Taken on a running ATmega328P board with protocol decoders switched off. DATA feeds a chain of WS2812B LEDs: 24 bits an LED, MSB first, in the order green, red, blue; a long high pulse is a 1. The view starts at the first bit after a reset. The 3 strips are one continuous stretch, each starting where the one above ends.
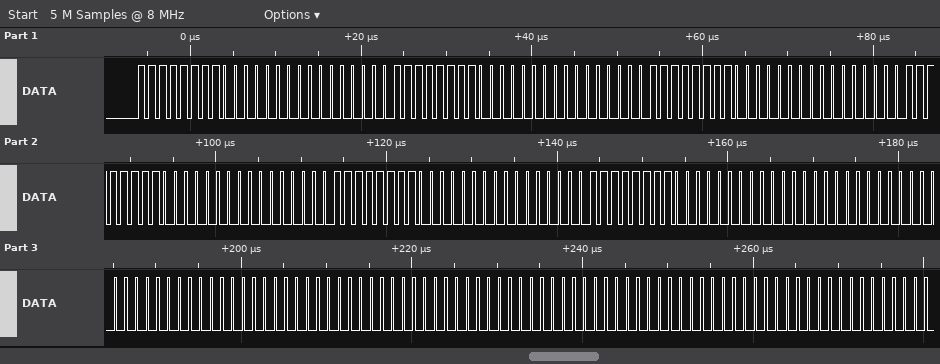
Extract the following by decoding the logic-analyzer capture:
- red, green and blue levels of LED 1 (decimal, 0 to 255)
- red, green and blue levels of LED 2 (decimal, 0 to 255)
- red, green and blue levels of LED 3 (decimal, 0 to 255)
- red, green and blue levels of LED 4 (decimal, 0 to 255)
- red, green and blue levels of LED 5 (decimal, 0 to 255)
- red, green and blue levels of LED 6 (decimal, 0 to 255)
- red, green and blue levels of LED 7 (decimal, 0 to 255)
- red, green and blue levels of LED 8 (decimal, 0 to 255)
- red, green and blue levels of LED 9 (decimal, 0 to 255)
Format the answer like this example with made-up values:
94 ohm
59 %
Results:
0, 255, 0
0, 255, 0
0, 255, 0
0, 255, 0
0, 255, 0
0, 255, 0
0, 0, 0
0, 0, 0
0, 0, 0
